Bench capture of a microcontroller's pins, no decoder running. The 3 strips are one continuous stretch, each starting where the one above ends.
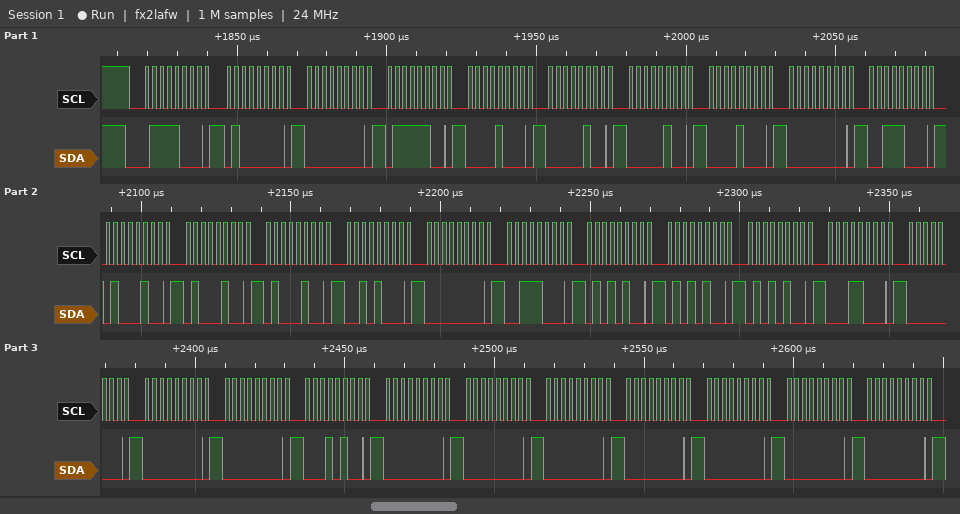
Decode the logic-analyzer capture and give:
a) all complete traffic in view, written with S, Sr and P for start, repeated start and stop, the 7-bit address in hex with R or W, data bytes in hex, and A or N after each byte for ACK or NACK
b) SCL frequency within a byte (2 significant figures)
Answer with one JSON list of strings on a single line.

["S 3CW A 40 A 00 A 7C A 08 A 04 A 04 A 08 A 00 A 38 A 44 A 44 A 44 A 28 A 00 A 38 A 54 A 54 A 54 A 18 A 00 A 00 A 00 A 14 A 00 A 00 A 00 A 00 A 00 A 00 A 00 A", "400 kHz"]
